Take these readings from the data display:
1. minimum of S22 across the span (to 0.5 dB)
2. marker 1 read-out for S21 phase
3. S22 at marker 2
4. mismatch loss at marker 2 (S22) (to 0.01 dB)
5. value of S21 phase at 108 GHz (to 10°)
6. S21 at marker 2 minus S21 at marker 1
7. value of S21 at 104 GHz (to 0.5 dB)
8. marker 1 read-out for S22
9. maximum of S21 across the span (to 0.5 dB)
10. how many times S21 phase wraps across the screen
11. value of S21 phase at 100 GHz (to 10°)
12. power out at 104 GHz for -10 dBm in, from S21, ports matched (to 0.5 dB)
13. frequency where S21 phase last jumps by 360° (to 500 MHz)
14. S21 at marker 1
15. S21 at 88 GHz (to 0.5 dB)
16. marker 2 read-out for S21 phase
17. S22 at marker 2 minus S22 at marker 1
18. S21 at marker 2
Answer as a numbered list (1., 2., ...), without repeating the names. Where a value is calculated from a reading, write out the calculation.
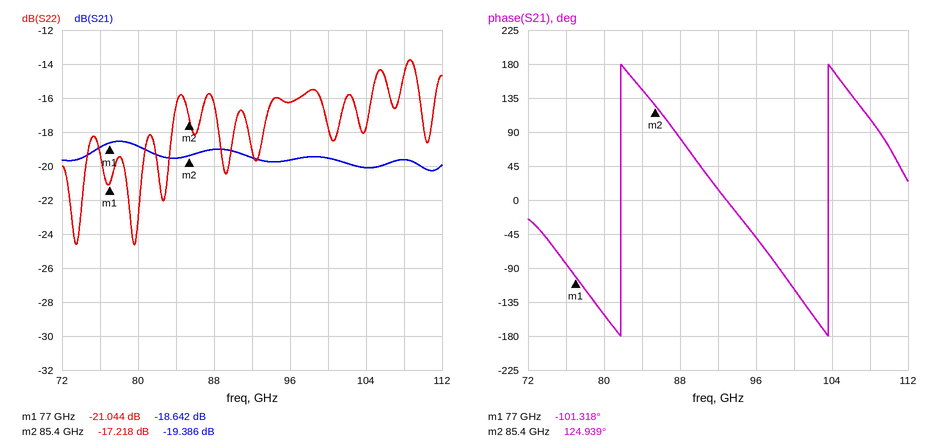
1. -24.5 dB
2. -101.318°
3. -17.218 dB
4. −10 log10(1 − 10^(-17.218/10)) ≈ 0.08 dB
5. 110°
6. -19.386 − (-18.642) = -0.744 dB
7. -20.0 dB
8. -21.044 dB
9. -18.5 dB
10. 2
11. -120°
12. -10 dBm + (-20.0 dB) = -30.0 dBm
13. 103.5 GHz
14. -18.642 dB
15. -19.0 dB
16. 124.939°
17. -17.218 − (-21.044) = 3.826 dB
18. -19.386 dB
